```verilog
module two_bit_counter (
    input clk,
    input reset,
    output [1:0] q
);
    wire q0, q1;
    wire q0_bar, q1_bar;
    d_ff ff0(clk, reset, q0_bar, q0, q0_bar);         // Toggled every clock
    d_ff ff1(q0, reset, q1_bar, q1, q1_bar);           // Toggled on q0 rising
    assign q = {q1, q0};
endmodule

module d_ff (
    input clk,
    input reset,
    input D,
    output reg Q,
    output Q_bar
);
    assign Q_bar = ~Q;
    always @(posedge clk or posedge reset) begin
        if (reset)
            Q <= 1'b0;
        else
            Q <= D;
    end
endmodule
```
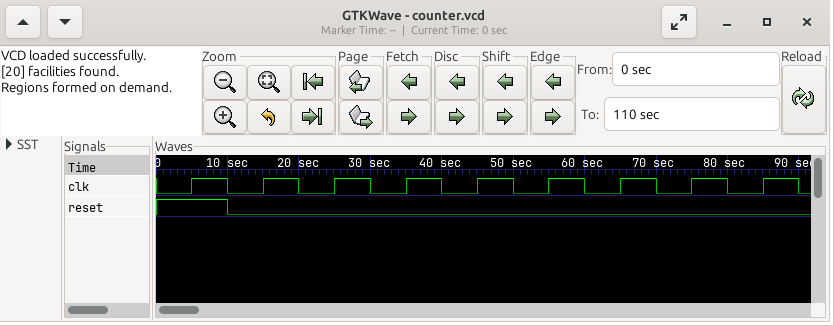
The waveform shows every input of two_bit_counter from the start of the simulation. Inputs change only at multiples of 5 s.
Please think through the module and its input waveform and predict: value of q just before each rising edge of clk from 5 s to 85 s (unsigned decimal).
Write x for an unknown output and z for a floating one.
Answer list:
0, 0, 3, 2, 1, 0, 3, 2, 1
